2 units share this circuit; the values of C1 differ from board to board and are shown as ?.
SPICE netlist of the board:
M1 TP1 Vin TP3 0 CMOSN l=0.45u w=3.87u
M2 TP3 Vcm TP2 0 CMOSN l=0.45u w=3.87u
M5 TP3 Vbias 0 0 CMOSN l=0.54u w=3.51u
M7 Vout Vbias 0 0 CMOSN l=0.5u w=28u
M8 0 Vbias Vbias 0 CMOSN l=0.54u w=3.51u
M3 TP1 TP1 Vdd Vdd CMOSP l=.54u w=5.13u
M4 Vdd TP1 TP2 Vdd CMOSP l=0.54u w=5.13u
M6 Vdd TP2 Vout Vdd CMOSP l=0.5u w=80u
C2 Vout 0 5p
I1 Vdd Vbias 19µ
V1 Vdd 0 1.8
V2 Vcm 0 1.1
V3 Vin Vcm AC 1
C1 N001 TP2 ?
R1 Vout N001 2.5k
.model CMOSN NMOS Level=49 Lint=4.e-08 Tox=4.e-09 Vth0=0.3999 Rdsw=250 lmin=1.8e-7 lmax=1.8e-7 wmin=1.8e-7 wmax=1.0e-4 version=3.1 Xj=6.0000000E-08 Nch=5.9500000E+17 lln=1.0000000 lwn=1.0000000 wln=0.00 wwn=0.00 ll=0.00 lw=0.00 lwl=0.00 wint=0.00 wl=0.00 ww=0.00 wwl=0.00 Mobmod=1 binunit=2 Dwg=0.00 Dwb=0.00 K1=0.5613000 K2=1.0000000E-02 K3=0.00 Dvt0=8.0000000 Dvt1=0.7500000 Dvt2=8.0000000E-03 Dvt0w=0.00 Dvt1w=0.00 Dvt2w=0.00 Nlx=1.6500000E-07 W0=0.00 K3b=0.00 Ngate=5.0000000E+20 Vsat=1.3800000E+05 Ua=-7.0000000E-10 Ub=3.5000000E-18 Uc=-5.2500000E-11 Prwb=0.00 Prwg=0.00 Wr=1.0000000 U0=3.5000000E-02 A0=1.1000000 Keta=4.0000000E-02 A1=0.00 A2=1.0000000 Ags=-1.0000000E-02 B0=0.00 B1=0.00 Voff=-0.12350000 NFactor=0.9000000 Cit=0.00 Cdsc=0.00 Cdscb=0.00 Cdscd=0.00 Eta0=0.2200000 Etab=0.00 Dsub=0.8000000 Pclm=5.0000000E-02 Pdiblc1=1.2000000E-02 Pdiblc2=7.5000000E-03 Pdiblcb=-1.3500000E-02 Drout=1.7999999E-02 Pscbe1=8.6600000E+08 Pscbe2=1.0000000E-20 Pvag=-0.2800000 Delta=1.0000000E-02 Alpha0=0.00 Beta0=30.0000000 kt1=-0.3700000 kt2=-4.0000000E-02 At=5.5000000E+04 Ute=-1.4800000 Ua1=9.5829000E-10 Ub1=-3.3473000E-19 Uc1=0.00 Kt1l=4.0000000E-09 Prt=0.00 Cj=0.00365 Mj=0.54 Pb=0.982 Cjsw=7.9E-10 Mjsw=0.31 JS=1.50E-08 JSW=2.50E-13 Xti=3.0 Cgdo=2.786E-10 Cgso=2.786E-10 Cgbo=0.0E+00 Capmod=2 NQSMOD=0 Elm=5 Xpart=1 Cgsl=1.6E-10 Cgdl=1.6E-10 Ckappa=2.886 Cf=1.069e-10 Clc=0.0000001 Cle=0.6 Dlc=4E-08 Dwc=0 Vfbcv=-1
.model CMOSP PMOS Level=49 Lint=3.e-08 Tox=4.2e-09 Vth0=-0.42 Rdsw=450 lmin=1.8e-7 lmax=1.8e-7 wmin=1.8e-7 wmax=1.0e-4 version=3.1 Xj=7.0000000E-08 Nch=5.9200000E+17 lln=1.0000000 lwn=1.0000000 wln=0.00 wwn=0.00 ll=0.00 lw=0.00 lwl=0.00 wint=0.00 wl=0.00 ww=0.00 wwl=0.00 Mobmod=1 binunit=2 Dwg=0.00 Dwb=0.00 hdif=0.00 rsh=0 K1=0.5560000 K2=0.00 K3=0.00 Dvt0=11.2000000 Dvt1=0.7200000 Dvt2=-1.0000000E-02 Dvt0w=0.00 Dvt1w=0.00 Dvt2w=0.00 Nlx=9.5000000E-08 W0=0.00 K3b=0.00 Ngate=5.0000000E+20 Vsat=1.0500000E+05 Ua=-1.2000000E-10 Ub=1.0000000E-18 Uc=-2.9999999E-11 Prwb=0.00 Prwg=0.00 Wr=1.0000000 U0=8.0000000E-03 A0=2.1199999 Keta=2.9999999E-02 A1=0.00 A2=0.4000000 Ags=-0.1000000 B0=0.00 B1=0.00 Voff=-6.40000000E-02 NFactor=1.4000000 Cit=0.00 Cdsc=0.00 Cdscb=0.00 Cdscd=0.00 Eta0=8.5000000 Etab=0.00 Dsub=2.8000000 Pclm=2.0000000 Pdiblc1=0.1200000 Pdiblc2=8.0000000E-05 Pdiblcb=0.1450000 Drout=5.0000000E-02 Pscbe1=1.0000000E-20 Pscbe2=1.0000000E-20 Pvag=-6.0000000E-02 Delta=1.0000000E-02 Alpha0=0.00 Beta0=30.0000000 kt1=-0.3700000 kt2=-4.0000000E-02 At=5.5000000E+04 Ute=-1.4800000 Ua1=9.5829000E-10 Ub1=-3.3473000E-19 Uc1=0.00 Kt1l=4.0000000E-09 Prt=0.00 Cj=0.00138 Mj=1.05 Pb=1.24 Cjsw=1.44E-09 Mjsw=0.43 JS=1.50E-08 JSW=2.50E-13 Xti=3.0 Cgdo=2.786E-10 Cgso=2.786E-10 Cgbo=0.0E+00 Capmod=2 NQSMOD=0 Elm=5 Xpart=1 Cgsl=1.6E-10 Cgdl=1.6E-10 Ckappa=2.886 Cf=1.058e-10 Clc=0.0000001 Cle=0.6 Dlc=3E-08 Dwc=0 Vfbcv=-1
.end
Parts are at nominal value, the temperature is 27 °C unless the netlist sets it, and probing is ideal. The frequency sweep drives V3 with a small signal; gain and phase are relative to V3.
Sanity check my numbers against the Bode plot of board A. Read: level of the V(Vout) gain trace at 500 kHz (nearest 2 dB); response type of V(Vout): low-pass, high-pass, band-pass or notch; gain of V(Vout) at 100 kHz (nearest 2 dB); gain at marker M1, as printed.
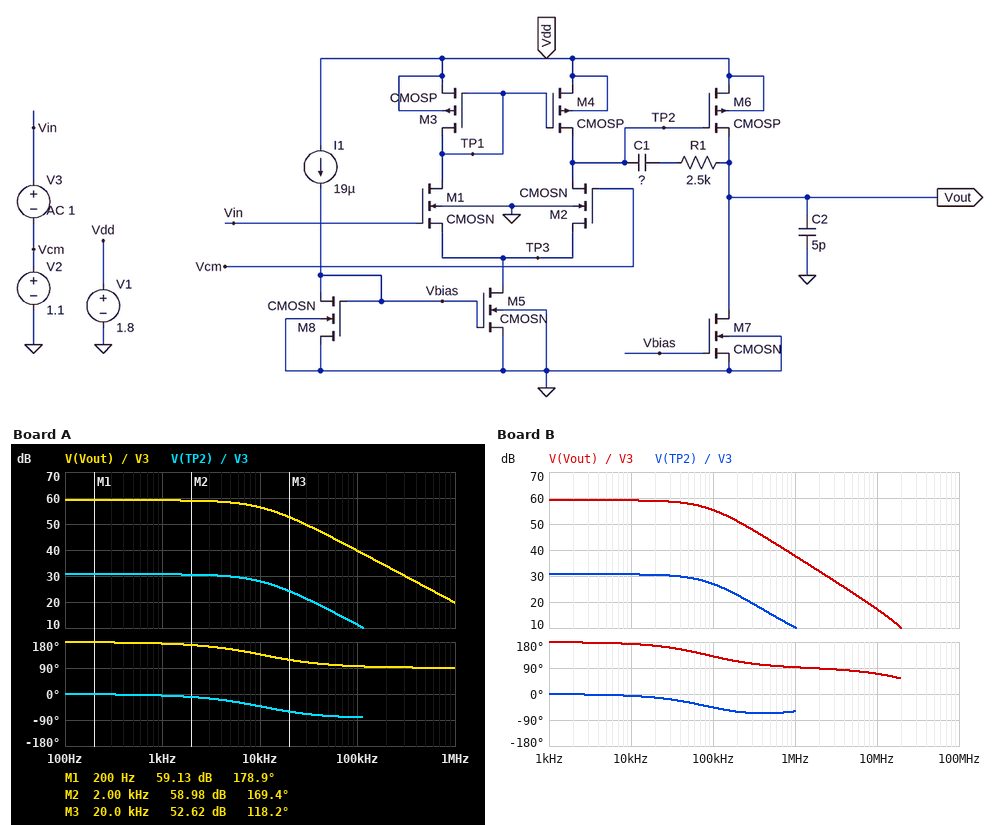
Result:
26 dB
low-pass
40 dB
59.13 dB
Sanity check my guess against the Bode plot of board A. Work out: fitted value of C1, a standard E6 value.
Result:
2.2 pF
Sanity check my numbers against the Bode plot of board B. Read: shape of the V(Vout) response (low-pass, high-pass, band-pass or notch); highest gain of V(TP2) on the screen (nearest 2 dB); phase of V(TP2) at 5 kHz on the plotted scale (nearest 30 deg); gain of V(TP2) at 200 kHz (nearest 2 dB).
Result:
low-pass
30 dB
0 deg
22 dB
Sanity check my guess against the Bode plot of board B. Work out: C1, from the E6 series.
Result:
220 fF
